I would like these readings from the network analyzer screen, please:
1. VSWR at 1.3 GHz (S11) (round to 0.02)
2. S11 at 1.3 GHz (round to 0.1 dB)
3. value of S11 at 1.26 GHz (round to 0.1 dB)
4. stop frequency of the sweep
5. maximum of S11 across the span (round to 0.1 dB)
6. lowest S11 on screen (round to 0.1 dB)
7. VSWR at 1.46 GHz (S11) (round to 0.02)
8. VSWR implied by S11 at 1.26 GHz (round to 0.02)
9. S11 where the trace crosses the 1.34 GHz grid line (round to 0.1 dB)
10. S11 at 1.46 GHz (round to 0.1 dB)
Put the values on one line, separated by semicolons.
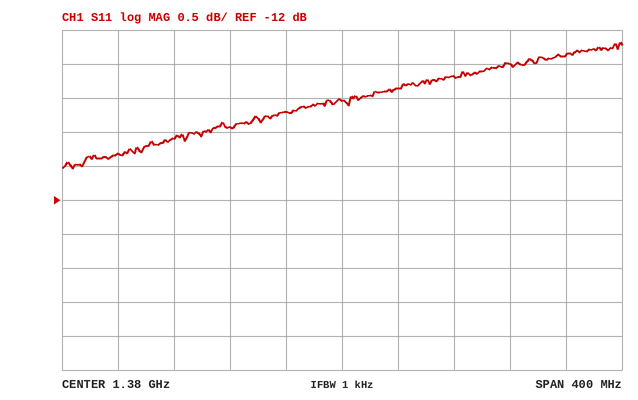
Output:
1.80; -10.9 dB; -11.1 dB; 1.58 GHz; -9.7 dB; -11.5 dB; 1.90; 1.78; -10.7 dB; -10.2 dB
